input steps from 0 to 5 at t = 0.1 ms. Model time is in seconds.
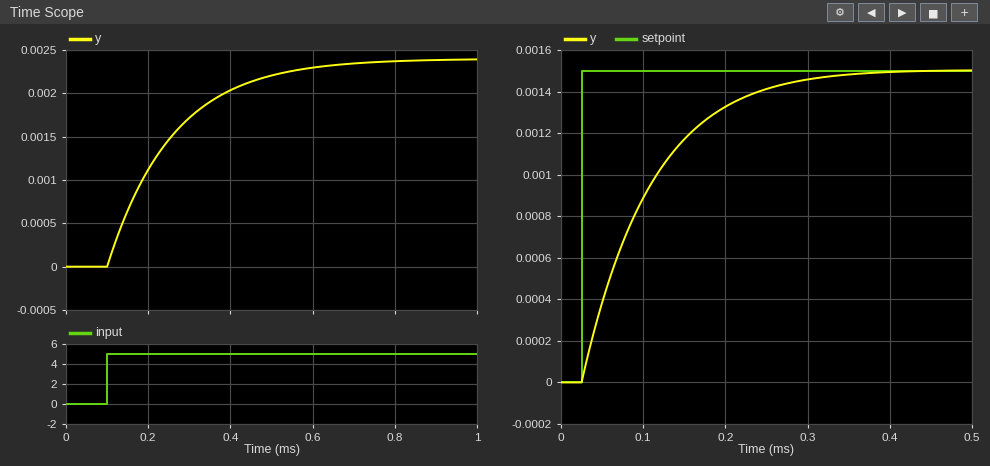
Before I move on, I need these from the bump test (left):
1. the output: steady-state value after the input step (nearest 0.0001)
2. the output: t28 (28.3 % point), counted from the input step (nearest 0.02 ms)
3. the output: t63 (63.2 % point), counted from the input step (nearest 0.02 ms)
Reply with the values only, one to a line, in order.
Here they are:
0.0024
0.06 ms
0.16 ms
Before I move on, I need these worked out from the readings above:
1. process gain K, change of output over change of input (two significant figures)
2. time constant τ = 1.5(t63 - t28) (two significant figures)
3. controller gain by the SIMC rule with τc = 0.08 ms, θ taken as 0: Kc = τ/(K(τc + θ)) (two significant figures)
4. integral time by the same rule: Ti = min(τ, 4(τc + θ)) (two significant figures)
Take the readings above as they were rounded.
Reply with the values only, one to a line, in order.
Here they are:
0.00048
0.15 ms
3900
0.15 ms
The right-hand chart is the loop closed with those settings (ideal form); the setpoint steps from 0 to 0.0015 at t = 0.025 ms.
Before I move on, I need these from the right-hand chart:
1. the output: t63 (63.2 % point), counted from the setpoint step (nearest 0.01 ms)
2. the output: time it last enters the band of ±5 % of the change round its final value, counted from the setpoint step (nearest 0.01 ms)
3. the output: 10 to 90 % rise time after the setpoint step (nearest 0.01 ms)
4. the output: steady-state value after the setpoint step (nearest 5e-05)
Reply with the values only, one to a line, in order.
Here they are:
0.08 ms
0.24 ms
0.18 ms
0.00150
